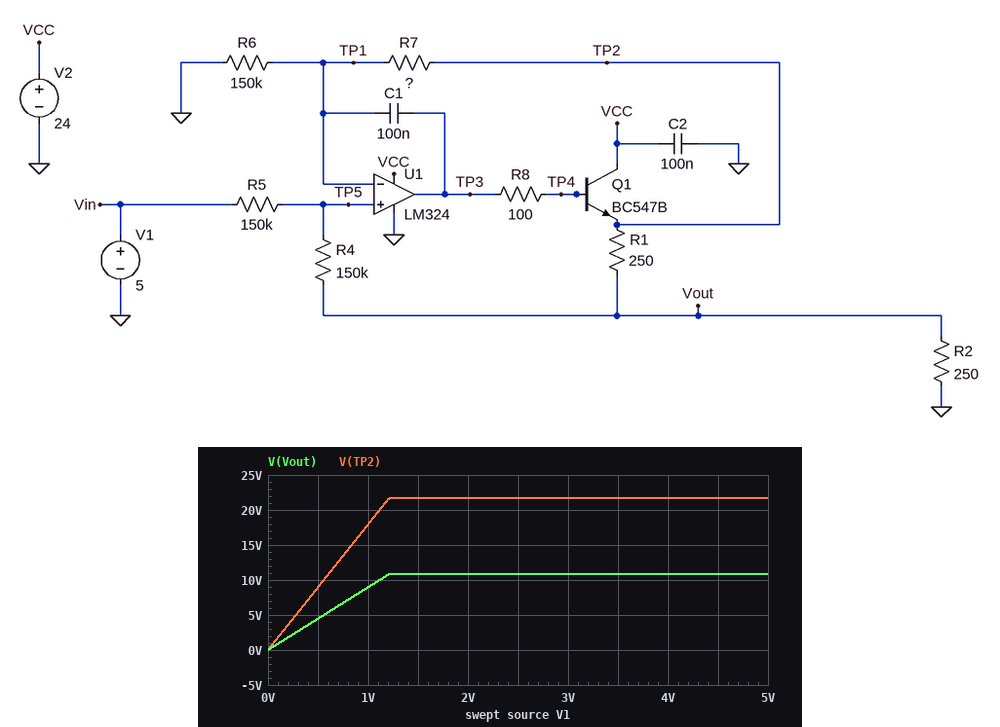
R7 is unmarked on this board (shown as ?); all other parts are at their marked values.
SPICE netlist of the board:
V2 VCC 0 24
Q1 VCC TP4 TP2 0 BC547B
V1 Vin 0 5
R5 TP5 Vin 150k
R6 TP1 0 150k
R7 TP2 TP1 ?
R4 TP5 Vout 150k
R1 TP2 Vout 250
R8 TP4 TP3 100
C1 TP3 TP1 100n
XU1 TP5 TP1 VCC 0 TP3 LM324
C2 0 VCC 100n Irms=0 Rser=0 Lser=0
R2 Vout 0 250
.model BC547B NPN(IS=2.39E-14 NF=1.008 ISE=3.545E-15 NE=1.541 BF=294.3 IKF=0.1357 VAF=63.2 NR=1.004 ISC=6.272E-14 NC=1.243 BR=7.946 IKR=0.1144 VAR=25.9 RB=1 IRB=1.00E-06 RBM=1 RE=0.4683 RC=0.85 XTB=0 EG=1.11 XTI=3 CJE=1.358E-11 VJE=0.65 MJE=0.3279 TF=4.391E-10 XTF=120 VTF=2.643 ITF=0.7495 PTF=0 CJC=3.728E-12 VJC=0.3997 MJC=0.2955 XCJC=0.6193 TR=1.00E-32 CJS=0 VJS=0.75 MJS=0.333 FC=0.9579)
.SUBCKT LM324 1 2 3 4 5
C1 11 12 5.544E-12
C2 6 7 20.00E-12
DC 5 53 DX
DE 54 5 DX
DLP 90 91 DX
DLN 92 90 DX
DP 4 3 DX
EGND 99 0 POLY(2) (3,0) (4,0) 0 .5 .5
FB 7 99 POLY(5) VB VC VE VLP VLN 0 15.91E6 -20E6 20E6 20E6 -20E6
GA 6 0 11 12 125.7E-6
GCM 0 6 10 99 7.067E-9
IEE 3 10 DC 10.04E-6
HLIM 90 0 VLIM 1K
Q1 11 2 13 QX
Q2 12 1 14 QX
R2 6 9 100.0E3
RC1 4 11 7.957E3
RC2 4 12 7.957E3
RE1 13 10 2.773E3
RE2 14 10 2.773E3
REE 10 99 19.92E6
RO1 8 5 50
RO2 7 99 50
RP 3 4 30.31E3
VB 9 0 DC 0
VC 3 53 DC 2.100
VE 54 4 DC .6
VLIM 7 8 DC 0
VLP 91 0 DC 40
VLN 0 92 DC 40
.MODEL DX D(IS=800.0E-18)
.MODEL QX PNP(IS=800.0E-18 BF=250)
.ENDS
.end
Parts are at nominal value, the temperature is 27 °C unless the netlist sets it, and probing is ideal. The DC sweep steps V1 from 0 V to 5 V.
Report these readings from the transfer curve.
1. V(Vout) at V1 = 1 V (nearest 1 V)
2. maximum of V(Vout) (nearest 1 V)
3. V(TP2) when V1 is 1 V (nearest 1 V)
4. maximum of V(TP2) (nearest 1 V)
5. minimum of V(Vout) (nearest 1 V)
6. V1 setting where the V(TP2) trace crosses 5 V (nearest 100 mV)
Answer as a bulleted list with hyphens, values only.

- 9 V
- 11 V
- 18 V
- 22 V
- 0 V
- 300 mV
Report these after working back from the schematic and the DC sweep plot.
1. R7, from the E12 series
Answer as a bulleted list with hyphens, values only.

- 390 kΩ
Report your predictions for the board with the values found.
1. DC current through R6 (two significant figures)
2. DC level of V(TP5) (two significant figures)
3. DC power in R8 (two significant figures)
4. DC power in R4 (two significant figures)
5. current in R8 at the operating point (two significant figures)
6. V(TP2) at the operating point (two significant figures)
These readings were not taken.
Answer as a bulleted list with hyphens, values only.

- 40 µA
- 7.9 V
- 3.8 µW
- 57 µW
- 200 µA
- 22 V
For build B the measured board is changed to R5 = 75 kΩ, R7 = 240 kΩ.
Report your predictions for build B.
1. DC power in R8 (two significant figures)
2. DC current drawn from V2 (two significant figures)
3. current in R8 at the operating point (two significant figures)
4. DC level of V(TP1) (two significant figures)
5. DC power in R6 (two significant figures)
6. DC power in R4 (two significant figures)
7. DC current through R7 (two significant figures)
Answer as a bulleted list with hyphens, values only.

- 1.3 µW
- 31 mA
- 110 µA
- 5.9 V
- 230 µW
- 21 µW
- 39 µA
